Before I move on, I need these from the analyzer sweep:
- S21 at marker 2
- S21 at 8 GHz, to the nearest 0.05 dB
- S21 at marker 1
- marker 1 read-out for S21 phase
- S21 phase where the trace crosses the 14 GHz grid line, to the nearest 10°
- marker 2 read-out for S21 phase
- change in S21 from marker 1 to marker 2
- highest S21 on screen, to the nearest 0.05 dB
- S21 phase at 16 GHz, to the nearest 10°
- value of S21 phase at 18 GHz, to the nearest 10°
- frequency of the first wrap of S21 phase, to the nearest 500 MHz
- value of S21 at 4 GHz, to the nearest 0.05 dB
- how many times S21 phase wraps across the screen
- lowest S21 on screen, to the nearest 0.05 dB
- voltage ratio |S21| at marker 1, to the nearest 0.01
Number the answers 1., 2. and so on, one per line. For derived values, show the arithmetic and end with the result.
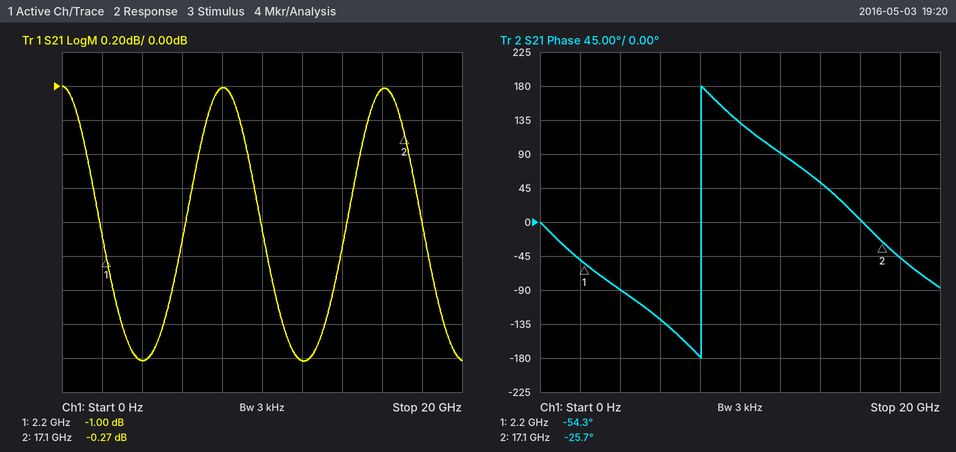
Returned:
1. -0.27 dB
2. 0.00 dB
3. -1.00 dB
4. -54.3°
5. 50°
6. -25.7°
7. -0.27 − (-1) = 0.73 dB
8. 0.00 dB
9. 0°
10. -50°
11. 8.0 GHz
12. -1.60 dB
13. 1
14. -1.60 dB
15. 10^(-1/20) ≈ 0.89
